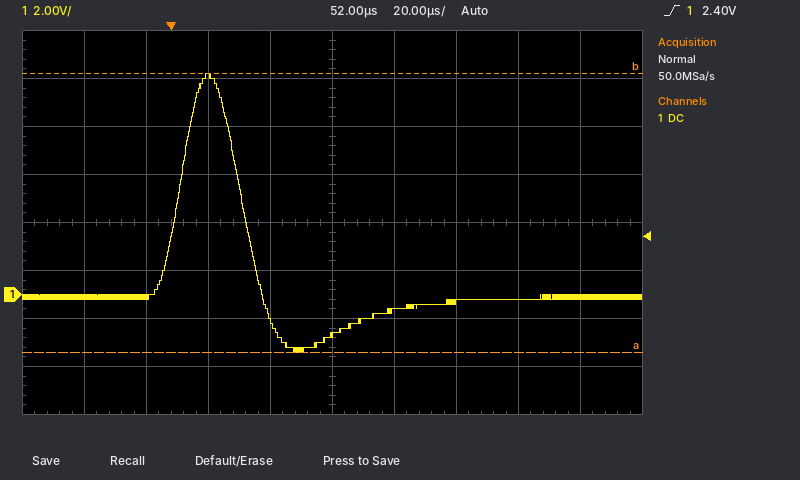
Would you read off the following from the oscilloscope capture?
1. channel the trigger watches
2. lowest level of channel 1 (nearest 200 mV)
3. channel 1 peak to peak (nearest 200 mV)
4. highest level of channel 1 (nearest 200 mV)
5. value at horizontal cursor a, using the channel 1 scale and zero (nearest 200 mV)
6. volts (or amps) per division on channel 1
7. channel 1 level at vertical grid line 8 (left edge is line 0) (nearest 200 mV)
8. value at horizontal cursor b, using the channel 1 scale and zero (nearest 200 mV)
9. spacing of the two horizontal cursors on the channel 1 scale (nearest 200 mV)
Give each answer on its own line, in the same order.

channel 1
-2.4 V
11.6 V
9.2 V
-2.4 V
2 V
-200 mV
9.2 V
11.6 V
